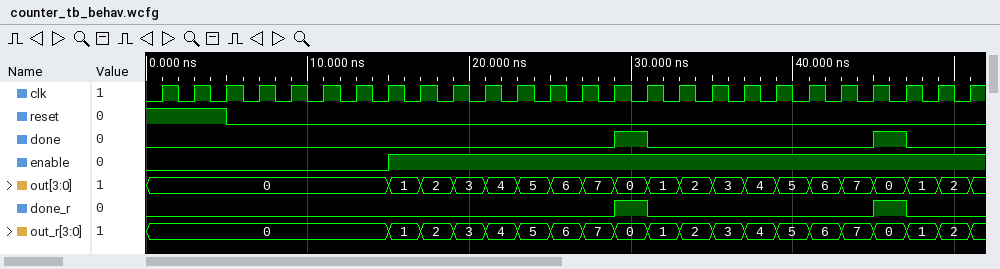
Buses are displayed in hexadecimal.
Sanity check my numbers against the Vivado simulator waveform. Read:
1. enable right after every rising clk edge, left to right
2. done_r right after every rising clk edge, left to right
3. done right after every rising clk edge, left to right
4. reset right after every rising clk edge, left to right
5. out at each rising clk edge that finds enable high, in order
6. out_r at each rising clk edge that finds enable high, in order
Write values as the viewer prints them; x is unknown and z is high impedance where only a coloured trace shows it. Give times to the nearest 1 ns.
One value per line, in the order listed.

0 0 0 0 0 0 0 1 1 1 1 1 1 1 1 1 1 1 1 1 1 1 1 1 1 1
0 0 0 0 0 0 0 0 0 0 0 0 0 0 1 0 0 0 0 0 0 0 1 0 0 0
0 0 0 0 0 0 0 0 0 0 0 0 0 0 1 0 0 0 0 0 0 0 1 0 0 0
1 1 0 0 0 0 0 0 0 0 0 0 0 0 0 0 0 0 0 0 0 0 0 0 0 0
1, 2, 3, 4, 5, 6, 7, 0, 1, 2, 3, 4, 5, 6, 7, 0, 1, 2
1, 2, 3, 4, 5, 6, 7, 0, 1, 2, 3, 4, 5, 6, 7, 0, 1, 2
